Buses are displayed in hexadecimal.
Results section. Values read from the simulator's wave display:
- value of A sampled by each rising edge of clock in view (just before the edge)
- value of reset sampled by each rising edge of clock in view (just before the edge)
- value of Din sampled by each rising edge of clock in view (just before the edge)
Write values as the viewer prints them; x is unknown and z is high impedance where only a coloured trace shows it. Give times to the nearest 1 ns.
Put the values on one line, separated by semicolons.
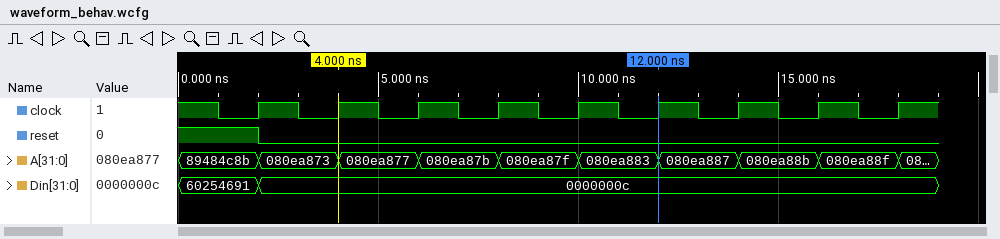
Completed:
89484c8b, 080ea873, 080ea877, 080ea87b, 080ea87f, 080ea883, 080ea887, 080ea88b, 080ea88f; 1 0 0 0 0 0 0 0 0; 60254691, 0000000c, 0000000c, 0000000c, 0000000c, 0000000c, 0000000c, 0000000c, 0000000c
